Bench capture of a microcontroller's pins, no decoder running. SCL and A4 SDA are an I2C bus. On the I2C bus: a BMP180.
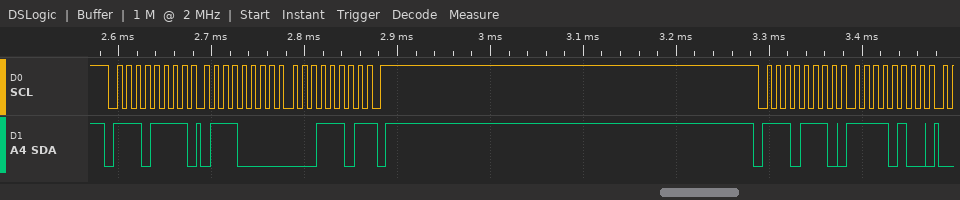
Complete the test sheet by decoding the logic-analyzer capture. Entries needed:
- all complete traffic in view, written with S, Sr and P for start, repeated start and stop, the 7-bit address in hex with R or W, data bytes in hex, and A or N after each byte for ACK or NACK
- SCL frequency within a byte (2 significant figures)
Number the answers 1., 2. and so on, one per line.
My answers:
1. S 77R A 70 A 1D N P S 77W A F4 A
2. 100 kHz
